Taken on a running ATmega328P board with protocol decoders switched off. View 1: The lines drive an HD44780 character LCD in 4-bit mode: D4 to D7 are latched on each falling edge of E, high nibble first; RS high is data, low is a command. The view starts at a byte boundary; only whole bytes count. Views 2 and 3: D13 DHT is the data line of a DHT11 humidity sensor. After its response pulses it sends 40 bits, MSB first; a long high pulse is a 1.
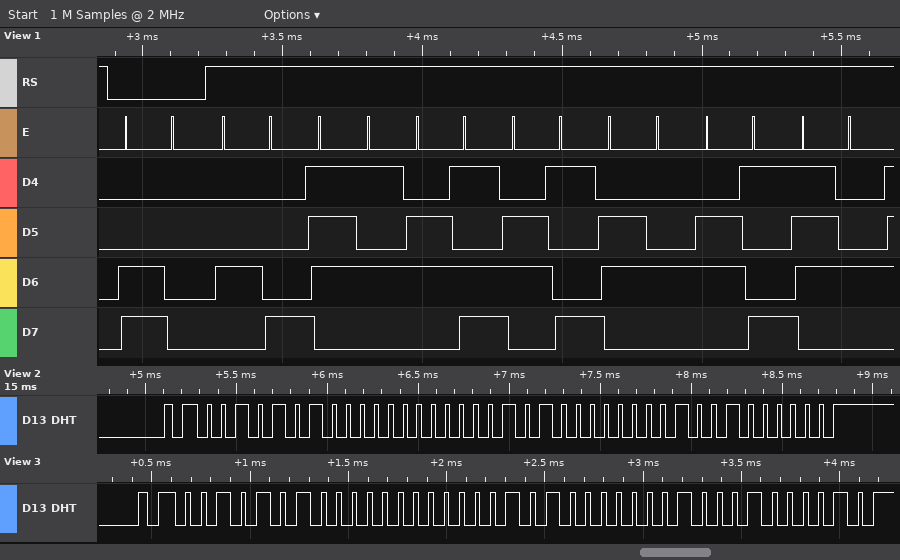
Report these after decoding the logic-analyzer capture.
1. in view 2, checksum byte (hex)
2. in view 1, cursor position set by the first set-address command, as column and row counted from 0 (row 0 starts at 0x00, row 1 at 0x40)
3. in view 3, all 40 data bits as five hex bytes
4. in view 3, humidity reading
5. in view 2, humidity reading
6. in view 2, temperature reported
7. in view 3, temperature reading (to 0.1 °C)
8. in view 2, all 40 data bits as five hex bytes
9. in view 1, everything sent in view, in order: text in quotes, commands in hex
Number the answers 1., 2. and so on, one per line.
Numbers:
1. 0x40
2. column 0, row 1
3. 2A 00 14 04 42
4. 42 %
5. 42 %
6. 20.2 °C
7. 20.4 °C
8. 2A 00 14 02 40
9. 0xC0 "Humidit"
